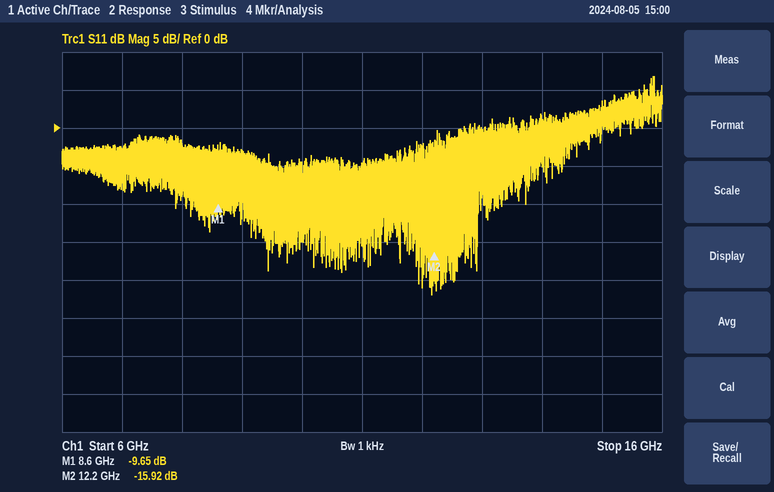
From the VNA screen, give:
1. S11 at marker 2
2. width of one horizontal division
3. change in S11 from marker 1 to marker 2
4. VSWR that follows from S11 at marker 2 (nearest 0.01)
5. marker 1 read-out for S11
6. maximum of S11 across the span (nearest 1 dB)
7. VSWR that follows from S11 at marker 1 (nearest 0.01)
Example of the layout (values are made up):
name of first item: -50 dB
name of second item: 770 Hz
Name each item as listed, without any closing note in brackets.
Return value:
S11 at marker 2: -15.92 dB
width of one horizontal division: 1 GHz
change in S11 from marker 1 to marker 2: -6.27 dB
VSWR that follows from S11 at marker 2: 1.38
marker 1 read-out for S11: -9.65 dB
maximum of S11 across the span: 7 dB
VSWR that follows from S11 at marker 1: 1.98
